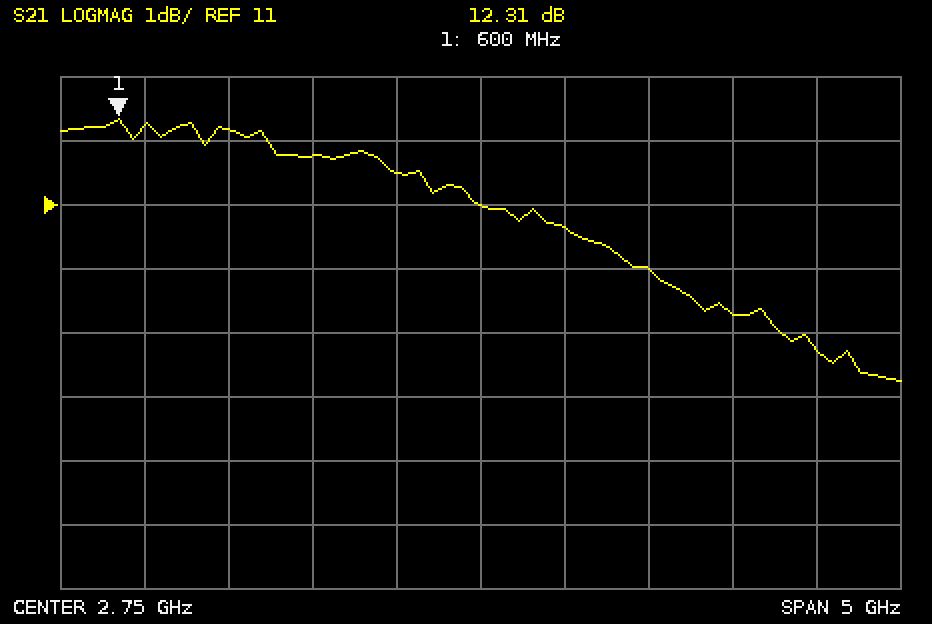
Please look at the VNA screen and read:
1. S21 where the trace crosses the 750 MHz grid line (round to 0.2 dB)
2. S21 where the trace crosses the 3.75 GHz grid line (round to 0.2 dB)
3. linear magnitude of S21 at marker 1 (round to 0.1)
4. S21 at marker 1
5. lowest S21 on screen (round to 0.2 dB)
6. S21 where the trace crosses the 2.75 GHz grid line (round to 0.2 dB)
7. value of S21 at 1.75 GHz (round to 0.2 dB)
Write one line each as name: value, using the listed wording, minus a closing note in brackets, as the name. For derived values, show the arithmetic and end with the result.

S21 where the trace crosses the 750 MHz grid line: 12.2 dB
S21 where the trace crosses the 3.75 GHz grid line: 10.0 dB
linear magnitude of S21 at marker 1: 10^(12.31/20) ≈ 4.1
S21 at marker 1: 12.31 dB
lowest S21 on screen: 8.2 dB
S21 where the trace crosses the 2.75 GHz grid line: 11.0 dB
value of S21 at 1.75 GHz: 11.8 dB
